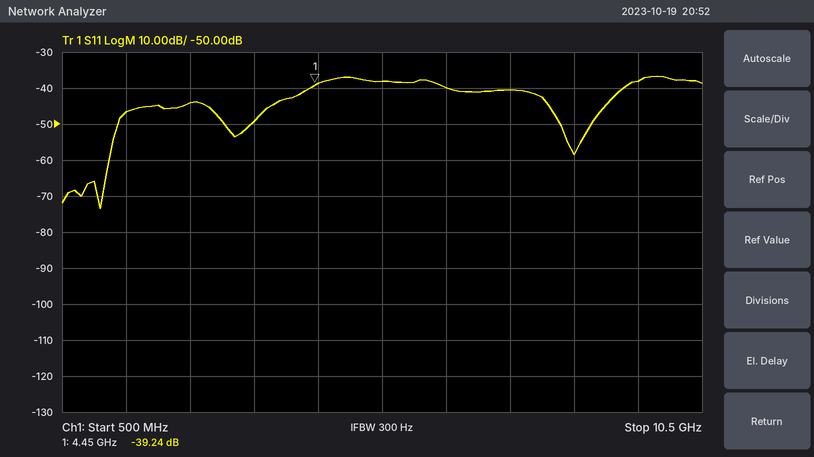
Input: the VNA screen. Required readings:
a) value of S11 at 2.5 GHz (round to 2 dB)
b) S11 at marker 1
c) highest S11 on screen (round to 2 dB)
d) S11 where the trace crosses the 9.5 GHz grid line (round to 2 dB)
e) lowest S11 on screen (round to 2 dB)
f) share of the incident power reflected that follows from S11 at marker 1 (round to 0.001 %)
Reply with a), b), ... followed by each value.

a) -44 dB
b) -39.24 dB
c) -36 dB
d) -38 dB
e) -74 dB
f) 0.012 %
